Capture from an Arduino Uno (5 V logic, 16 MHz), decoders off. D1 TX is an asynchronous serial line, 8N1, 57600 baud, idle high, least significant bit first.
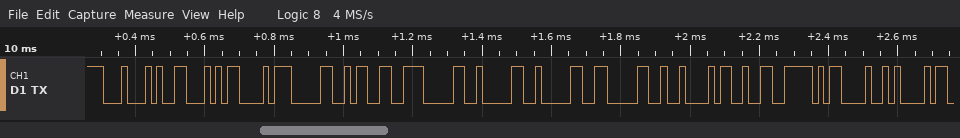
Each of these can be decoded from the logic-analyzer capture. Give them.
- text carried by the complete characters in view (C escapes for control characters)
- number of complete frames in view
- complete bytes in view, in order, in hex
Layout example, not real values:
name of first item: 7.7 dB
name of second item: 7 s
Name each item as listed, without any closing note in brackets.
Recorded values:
text carried by the complete characters in view: "DFC030000B2\r\n"
number of complete frames in view: 13
complete bytes in view, in order, in hex: 0x44 0x46 0x43 0x30 0x33 0x30 0x30 0x30 0x30 0x42 0x32 0x0D 0x0A
